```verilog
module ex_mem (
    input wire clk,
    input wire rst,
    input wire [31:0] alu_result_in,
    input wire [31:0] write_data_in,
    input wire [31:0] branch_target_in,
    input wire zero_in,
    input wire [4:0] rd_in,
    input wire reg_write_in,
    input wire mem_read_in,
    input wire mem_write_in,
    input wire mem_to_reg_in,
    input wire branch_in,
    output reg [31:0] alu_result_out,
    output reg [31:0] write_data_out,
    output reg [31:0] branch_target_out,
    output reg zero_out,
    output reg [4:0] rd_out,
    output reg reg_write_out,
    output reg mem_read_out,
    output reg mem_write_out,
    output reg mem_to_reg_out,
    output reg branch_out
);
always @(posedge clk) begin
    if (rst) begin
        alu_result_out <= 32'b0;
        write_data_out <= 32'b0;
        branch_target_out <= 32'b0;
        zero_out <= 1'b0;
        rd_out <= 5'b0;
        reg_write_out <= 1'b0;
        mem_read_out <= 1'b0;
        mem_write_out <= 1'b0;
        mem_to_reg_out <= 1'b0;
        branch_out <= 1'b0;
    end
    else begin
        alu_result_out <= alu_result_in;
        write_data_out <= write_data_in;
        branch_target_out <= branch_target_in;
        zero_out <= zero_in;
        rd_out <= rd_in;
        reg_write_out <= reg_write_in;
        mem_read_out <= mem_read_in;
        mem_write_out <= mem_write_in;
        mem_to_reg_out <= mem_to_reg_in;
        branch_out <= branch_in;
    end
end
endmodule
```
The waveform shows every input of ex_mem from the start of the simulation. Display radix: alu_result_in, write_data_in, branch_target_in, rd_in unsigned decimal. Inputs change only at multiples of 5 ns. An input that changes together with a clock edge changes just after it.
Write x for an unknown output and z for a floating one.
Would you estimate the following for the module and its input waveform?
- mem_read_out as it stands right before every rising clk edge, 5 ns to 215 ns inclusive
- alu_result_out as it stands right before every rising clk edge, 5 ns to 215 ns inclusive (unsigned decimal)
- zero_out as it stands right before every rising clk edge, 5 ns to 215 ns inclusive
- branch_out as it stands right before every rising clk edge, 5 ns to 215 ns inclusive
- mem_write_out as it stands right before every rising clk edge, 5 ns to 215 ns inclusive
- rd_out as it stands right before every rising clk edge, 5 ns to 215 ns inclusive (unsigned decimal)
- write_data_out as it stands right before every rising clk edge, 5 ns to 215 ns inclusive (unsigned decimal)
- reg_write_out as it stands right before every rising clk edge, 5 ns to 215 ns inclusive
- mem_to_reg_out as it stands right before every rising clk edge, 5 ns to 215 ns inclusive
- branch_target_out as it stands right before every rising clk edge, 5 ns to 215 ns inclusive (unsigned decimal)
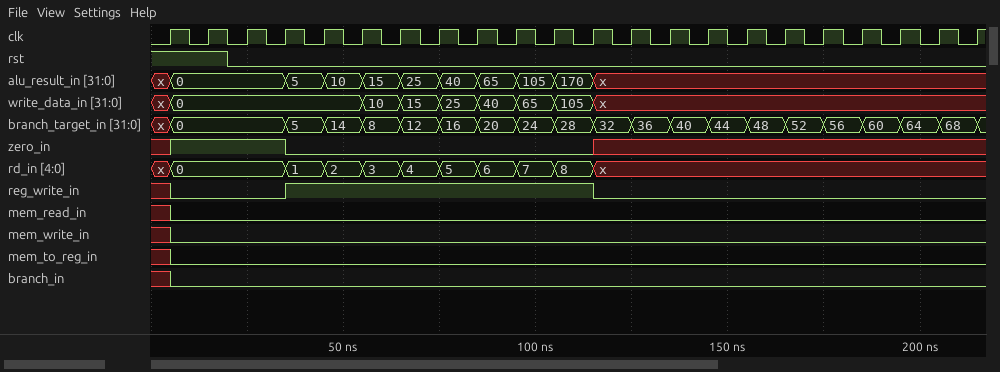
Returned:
x 0 0 0 0 0 0 0 0 0 0 0 0 0 0 0 0 0 0 0 0 0
x, 0, 0, 0, 0, 5, 10, 15, 25, 40, 65, 105, 170, x, x, x, x, x, x, x, x, x
x 0 0 1 1 0 0 0 0 0 0 0 0 x x x x x x x x x
x 0 0 0 0 0 0 0 0 0 0 0 0 0 0 0 0 0 0 0 0 0
x 0 0 0 0 0 0 0 0 0 0 0 0 0 0 0 0 0 0 0 0 0
x, 0, 0, 0, 0, 1, 2, 3, 4, 5, 6, 7, 8, x, x, x, x, x, x, x, x, x
x, 0, 0, 0, 0, 0, 0, 10, 15, 25, 40, 65, 105, x, x, x, x, x, x, x, x, x
x 0 0 0 0 1 1 1 1 1 1 1 1 0 0 0 0 0 0 0 0 0
x 0 0 0 0 0 0 0 0 0 0 0 0 0 0 0 0 0 0 0 0 0
x, 0, 0, 0, 0, 5, 14, 8, 12, 16, 20, 24, 28, 32, 36, 40, 44, 48, 52, 56, 60, 64
